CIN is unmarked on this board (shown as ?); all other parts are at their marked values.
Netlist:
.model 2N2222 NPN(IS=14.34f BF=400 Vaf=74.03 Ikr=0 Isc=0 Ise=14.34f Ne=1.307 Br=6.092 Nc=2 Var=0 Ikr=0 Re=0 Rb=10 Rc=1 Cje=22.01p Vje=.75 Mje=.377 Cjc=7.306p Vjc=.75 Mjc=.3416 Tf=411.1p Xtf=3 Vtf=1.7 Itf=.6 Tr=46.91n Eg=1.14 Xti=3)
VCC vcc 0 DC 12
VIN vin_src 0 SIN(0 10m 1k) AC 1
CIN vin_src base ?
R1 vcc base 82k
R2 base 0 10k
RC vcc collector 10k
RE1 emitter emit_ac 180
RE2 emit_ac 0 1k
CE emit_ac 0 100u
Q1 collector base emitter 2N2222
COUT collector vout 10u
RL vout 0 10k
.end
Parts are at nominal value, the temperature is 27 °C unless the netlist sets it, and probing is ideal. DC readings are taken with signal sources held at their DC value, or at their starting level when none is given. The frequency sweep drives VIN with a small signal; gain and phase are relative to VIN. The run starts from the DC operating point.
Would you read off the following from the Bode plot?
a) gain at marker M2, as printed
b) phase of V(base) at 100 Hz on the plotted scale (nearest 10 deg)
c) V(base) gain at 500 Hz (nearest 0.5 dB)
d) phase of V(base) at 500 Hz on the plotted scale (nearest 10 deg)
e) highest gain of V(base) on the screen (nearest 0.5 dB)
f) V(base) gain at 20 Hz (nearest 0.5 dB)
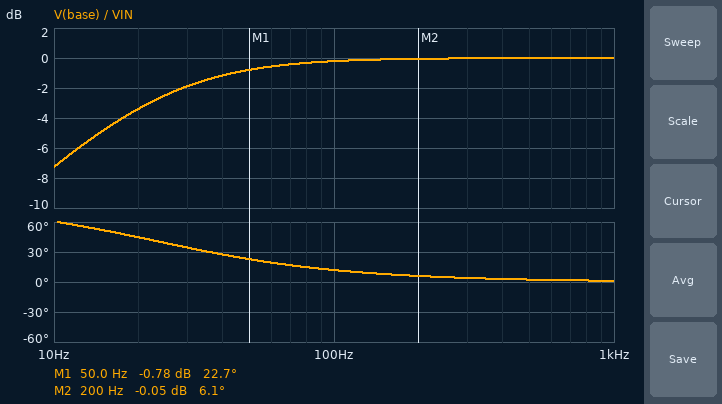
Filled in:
-0.05 dB
10 deg
0 dB
0 deg
0 dB
-3.5 dB
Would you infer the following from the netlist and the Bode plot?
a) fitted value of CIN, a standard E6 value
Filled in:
1 µF
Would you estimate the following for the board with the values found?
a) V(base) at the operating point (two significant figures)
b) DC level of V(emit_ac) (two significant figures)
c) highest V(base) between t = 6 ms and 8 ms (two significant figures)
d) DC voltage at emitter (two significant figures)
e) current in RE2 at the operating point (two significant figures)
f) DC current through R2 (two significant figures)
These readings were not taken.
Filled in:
1.3 V
550 mV
1.3 V
650 mV
550 µA
130 µA
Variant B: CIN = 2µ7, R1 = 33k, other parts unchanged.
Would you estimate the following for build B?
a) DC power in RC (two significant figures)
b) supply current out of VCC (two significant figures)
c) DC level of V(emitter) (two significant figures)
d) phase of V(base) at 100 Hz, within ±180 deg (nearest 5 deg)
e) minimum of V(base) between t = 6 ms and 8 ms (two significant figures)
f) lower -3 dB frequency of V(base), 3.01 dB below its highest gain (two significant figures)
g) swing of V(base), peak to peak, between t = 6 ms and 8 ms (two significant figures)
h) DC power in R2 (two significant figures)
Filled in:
11 mW
1.4 mA
1.4 V
60 deg
2.0 V
210 Hz
20 mV
410 µW
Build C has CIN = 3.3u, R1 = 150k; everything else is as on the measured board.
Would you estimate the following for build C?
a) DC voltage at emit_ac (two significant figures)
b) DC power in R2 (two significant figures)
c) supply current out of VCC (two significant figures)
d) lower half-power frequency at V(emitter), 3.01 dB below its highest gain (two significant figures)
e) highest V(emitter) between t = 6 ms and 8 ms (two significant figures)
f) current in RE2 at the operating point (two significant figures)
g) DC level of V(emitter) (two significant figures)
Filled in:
130 mV
55 µW
200 µA
2.8 Hz
160 mV
130 µA
150 mV
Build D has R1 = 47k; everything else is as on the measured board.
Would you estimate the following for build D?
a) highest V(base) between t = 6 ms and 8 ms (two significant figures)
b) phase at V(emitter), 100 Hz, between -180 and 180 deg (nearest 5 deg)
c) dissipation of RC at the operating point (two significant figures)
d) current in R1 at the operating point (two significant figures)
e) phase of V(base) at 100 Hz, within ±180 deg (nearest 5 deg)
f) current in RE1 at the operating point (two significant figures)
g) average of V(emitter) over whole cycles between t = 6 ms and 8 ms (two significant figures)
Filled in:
1.9 V
70 deg
11 mW
210 µA
75 deg
1.1 mA
1.3 V
